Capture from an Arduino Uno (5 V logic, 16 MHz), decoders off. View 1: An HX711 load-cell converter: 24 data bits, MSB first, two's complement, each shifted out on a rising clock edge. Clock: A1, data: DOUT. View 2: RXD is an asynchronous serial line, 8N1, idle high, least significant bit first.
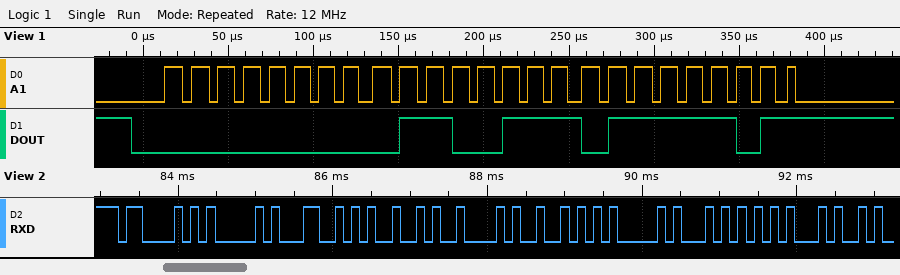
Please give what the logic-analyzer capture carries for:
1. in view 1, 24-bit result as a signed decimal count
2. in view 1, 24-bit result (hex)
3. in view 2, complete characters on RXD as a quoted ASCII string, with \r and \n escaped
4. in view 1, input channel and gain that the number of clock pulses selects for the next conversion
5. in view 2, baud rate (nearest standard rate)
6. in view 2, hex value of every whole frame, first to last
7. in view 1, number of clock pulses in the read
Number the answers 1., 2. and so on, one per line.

1. 26493
2. 0x00677D
3. "CALIBRATE"
4. channel A, gain 128
5. 9600 baud
6. 43 41 4C 49 42 52 41 54 45
7. 25
